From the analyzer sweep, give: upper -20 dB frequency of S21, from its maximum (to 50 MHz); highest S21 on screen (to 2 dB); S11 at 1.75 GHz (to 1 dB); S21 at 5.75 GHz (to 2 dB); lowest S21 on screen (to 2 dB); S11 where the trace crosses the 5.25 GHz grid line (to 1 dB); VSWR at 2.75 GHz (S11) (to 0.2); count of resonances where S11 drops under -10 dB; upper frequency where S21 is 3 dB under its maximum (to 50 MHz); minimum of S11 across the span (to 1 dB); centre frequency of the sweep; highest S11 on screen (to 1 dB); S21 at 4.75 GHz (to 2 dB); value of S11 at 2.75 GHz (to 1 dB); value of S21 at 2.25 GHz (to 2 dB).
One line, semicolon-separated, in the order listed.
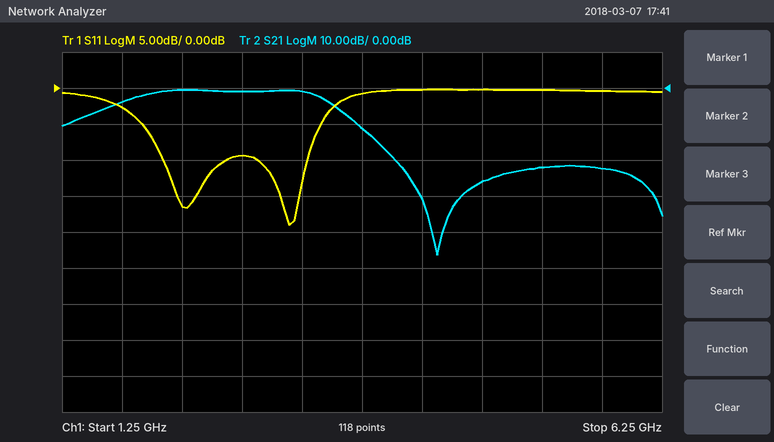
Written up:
4.05 GHz; 0 dB; -3 dB; -22 dB; -46 dB; 0 dB; 2.0; 2; 3.45 GHz; -19 dB; 3.75 GHz; 0 dB; -26 dB; -9 dB; 0 dB
